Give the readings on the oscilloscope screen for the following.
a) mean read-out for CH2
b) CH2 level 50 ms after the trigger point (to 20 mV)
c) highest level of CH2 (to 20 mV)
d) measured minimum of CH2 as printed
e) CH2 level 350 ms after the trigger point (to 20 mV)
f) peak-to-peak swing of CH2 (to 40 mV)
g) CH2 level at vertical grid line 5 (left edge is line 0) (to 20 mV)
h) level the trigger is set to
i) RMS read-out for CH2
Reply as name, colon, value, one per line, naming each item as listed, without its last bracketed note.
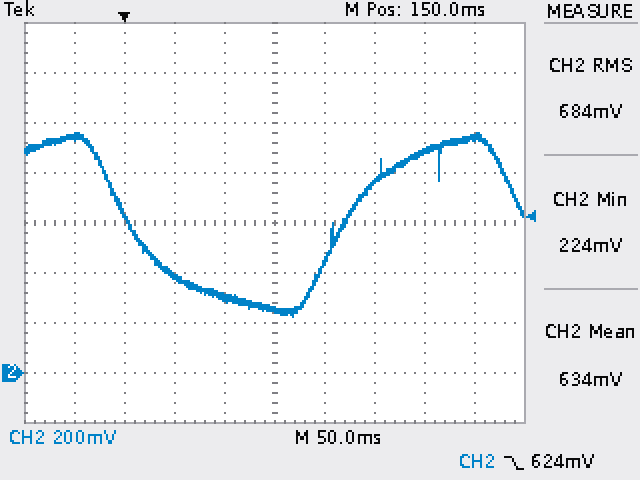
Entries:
mean read-out for CH2: 634 mV
CH2 level 50 ms after the trigger point: 380 mV
highest level of CH2: 960 mV
measured minimum of CH2 as printed: 224 mV
CH2 level 350 ms after the trigger point: 940 mV
peak-to-peak swing of CH2: 720 mV
CH2 level at vertical grid line 5 (left edge is line 0): 260 mV
level the trigger is set to: 624 mV
RMS read-out for CH2: 684 mV
